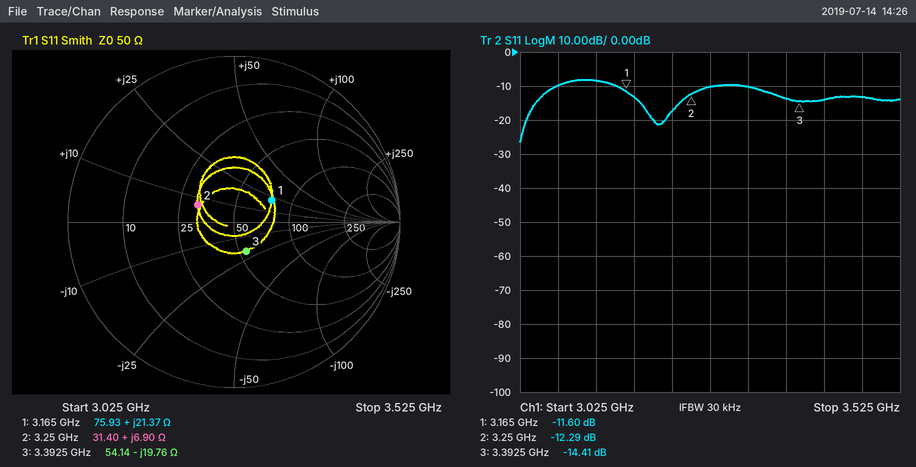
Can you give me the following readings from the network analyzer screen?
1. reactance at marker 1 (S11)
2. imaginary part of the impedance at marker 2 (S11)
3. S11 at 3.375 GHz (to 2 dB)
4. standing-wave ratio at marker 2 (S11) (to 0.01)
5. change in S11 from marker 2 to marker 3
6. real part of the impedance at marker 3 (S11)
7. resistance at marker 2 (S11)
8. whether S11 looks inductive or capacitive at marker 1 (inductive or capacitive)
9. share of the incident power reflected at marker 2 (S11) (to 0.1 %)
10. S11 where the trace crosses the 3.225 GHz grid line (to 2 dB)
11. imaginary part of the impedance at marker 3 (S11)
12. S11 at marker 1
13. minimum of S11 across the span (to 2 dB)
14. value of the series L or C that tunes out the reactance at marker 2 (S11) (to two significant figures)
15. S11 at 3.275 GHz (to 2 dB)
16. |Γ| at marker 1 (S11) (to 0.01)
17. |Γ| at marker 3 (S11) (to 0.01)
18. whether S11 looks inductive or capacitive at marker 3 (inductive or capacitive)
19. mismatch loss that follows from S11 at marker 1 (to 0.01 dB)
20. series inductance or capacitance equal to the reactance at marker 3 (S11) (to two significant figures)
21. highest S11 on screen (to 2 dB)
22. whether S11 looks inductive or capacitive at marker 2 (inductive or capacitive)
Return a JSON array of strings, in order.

["+21.37 Ω", "+6.90 Ω", "-14 dB", "1.64", "-2.12 dB", "54.14 Ω", "31.40 Ω", "inductive", "5.9 %", "-18 dB", "-19.76 Ω", "-11.60 dB", "-26 dB", "7.1 pF", "-10 dB", "0.26", "0.19", "capacitive", "0.31 dB", "2.4 pF", "-8 dB", "inductive"]
